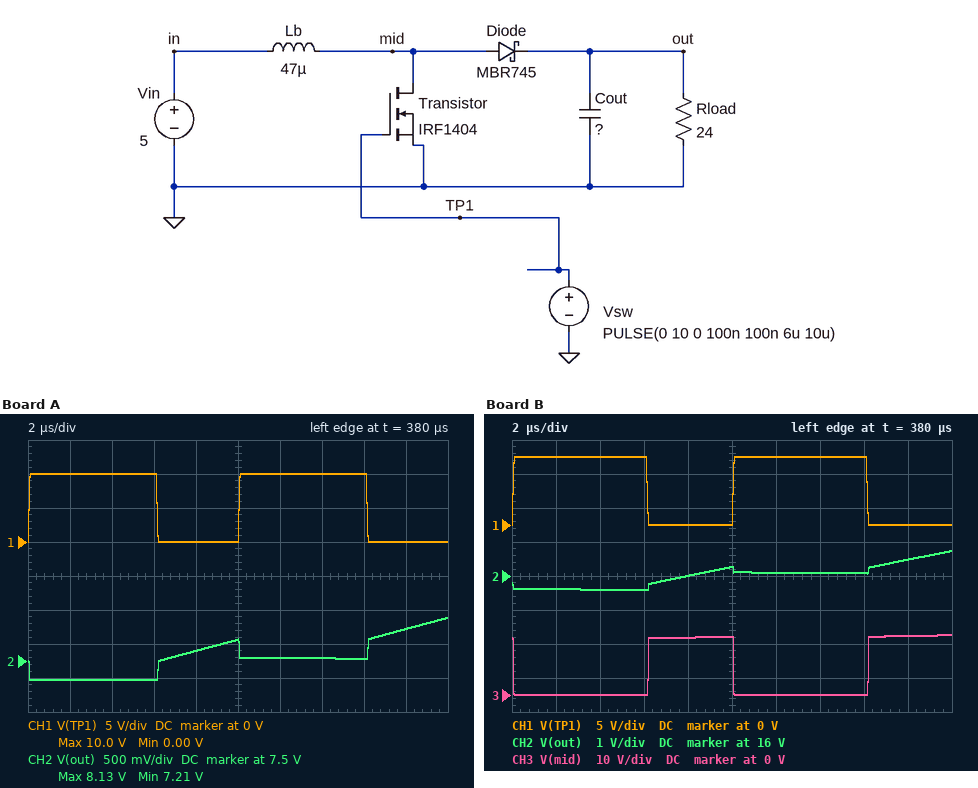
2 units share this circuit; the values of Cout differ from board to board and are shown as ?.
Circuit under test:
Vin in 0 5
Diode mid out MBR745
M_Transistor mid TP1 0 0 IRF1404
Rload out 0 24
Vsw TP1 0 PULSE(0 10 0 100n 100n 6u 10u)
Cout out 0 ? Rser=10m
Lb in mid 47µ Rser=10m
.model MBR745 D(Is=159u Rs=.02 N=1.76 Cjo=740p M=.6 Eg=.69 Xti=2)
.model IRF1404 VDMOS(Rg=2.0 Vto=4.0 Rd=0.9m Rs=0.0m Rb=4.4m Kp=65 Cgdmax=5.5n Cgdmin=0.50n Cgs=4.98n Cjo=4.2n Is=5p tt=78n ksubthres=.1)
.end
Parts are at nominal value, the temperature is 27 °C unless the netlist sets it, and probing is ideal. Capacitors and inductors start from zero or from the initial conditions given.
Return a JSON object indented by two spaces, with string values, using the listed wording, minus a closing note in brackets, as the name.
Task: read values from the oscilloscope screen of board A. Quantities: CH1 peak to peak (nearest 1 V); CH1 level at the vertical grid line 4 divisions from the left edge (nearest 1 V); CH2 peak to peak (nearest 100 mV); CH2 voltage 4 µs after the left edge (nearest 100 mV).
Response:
{
  "CH1 peak to peak": "10 V",
  "CH1 level at the vertical grid line 4 divisions from the left edge": "0 V",
  "CH2 peak to peak": "900 mV",
  "CH2 voltage 4 µs after the left edge": "7.2 V"
}
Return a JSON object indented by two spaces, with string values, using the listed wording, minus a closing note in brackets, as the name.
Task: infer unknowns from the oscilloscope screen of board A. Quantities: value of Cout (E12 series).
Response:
{
  "value of Cout": "330 µF"
}
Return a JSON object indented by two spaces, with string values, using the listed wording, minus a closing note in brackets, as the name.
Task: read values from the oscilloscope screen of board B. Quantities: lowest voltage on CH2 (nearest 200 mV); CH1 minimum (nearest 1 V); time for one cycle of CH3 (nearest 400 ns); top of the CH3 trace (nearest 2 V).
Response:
{
  "lowest voltage on CH2": "15.6 V",
  "CH1 minimum": "0 V",
  "time for one cycle of CH3": "10.0 µs",
  "top of the CH3 trace": "18 V"
}
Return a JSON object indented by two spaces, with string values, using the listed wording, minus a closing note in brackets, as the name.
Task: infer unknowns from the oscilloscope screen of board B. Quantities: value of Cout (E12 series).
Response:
{
  "value of Cout": "120 µF"
}
